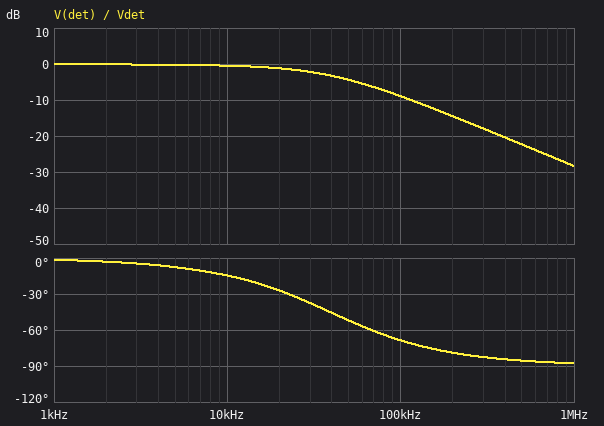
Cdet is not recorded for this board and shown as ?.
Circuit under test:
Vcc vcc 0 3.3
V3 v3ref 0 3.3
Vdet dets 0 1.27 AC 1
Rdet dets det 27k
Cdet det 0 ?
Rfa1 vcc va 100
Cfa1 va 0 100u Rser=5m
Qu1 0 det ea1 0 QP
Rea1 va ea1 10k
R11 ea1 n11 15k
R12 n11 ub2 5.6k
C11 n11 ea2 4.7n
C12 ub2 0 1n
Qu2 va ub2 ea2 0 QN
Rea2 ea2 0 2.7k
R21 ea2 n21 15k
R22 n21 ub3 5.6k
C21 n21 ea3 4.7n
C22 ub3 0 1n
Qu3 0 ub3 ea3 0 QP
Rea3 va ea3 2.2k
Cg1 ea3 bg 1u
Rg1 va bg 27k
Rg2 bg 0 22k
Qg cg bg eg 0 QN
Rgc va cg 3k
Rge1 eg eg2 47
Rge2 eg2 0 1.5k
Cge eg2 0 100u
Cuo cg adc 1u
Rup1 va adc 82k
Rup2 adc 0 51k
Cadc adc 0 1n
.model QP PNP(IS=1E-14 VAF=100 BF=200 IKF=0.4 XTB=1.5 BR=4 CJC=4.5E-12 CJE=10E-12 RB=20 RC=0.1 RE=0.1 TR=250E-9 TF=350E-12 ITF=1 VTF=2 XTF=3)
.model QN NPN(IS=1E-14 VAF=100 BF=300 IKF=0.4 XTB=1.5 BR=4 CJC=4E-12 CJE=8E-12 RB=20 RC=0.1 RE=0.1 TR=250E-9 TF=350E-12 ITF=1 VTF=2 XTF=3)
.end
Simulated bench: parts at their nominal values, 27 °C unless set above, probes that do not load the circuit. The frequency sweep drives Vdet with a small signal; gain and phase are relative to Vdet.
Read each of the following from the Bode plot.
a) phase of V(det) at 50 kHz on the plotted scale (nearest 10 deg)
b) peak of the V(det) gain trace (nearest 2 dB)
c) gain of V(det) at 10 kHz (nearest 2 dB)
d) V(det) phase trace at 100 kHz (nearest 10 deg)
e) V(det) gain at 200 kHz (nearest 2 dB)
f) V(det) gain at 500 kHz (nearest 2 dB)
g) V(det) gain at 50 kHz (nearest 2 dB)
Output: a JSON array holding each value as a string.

["-50 deg", "0 dB", "0 dB", "-70 deg", "-14 dB", "-22 dB", "-4 dB"]
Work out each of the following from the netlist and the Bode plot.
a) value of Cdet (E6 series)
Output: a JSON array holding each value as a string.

["150 pF"]
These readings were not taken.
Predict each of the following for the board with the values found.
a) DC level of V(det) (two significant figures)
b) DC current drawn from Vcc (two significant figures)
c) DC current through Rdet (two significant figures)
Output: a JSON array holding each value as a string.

["1.3 V", "1.7 mA", "600 nA"]
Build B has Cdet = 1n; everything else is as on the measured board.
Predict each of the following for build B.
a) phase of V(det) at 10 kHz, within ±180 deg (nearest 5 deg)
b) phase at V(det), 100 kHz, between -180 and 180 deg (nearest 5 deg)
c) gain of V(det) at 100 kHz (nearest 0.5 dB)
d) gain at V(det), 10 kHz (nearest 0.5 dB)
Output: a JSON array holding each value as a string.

["-60 deg", "-85 deg", "-24.5 dB", "-6.0 dB"]
